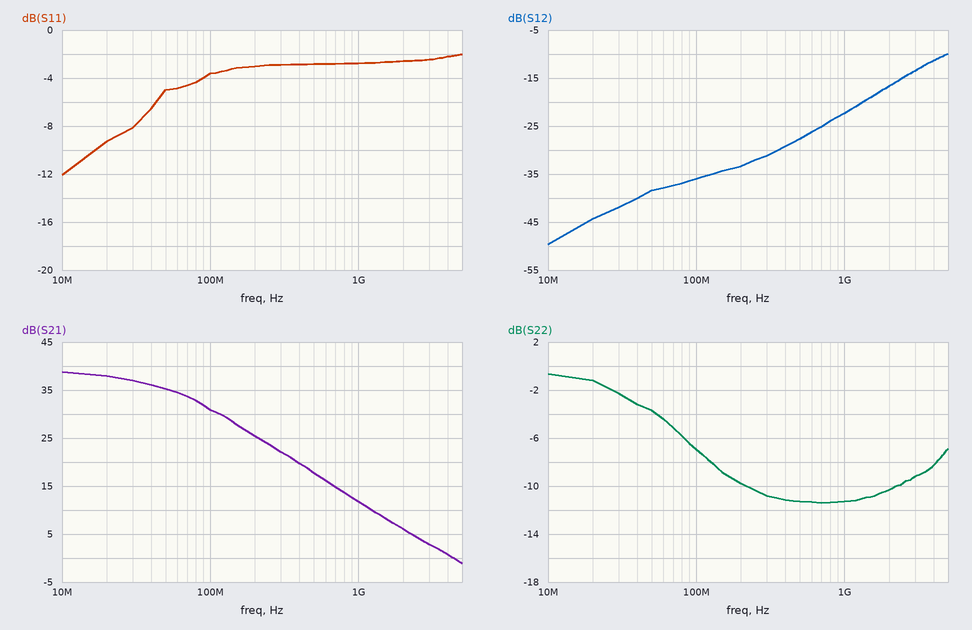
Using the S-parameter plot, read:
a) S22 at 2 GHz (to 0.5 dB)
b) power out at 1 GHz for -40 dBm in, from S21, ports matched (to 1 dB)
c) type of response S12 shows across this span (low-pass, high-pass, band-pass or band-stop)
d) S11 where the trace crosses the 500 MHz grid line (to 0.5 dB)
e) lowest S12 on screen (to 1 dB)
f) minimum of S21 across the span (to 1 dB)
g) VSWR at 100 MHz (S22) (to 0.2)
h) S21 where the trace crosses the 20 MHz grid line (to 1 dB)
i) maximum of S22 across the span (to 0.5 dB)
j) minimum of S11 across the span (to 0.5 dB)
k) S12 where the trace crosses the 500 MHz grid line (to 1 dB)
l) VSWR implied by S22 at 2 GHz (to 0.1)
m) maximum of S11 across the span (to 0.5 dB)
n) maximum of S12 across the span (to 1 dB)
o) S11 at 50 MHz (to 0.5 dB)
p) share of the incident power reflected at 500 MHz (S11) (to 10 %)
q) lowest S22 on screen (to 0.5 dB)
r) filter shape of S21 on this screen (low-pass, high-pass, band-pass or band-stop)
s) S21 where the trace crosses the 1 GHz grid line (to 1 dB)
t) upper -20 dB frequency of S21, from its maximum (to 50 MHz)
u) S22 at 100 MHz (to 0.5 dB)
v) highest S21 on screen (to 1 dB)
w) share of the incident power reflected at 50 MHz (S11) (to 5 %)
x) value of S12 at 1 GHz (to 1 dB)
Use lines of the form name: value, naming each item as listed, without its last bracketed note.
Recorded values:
S22 at 2 GHz: -10.5 dB
power out at 1 GHz for -40 dBm in, from S21, ports matched: -28 dBm
type of response S12 shows across this span: high-pass
S11 where the trace crosses the 500 MHz grid line: -3.0 dB
lowest S12 on screen: -50 dB
minimum of S21 across the span: -1 dB
VSWR at 100 MHz (S22): 2.6
S21 where the trace crosses the 20 MHz grid line: 38 dB
maximum of S22 across the span: -0.5 dB
minimum of S11 across the span: -12.0 dB
S12 where the trace crosses the 500 MHz grid line: -28 dB
VSWR implied by S22 at 2 GHz: 1.9
maximum of S11 across the span: -2.0 dB
maximum of S12 across the span: -10 dB
S11 at 50 MHz: -5.0 dB
share of the incident power reflected at 500 MHz (S11): 50 %
lowest S22 on screen: -11.5 dB
filter shape of S21 on this screen: low-pass
S21 where the trace crosses the 1 GHz grid line: 12 dB
upper -20 dB frequency of S21, from its maximum: 450 MHz
S22 at 100 MHz: -7.0 dB
highest S21 on screen: 39 dB
share of the incident power reflected at 50 MHz (S11): 30 %
value of S12 at 1 GHz: -22 dB
